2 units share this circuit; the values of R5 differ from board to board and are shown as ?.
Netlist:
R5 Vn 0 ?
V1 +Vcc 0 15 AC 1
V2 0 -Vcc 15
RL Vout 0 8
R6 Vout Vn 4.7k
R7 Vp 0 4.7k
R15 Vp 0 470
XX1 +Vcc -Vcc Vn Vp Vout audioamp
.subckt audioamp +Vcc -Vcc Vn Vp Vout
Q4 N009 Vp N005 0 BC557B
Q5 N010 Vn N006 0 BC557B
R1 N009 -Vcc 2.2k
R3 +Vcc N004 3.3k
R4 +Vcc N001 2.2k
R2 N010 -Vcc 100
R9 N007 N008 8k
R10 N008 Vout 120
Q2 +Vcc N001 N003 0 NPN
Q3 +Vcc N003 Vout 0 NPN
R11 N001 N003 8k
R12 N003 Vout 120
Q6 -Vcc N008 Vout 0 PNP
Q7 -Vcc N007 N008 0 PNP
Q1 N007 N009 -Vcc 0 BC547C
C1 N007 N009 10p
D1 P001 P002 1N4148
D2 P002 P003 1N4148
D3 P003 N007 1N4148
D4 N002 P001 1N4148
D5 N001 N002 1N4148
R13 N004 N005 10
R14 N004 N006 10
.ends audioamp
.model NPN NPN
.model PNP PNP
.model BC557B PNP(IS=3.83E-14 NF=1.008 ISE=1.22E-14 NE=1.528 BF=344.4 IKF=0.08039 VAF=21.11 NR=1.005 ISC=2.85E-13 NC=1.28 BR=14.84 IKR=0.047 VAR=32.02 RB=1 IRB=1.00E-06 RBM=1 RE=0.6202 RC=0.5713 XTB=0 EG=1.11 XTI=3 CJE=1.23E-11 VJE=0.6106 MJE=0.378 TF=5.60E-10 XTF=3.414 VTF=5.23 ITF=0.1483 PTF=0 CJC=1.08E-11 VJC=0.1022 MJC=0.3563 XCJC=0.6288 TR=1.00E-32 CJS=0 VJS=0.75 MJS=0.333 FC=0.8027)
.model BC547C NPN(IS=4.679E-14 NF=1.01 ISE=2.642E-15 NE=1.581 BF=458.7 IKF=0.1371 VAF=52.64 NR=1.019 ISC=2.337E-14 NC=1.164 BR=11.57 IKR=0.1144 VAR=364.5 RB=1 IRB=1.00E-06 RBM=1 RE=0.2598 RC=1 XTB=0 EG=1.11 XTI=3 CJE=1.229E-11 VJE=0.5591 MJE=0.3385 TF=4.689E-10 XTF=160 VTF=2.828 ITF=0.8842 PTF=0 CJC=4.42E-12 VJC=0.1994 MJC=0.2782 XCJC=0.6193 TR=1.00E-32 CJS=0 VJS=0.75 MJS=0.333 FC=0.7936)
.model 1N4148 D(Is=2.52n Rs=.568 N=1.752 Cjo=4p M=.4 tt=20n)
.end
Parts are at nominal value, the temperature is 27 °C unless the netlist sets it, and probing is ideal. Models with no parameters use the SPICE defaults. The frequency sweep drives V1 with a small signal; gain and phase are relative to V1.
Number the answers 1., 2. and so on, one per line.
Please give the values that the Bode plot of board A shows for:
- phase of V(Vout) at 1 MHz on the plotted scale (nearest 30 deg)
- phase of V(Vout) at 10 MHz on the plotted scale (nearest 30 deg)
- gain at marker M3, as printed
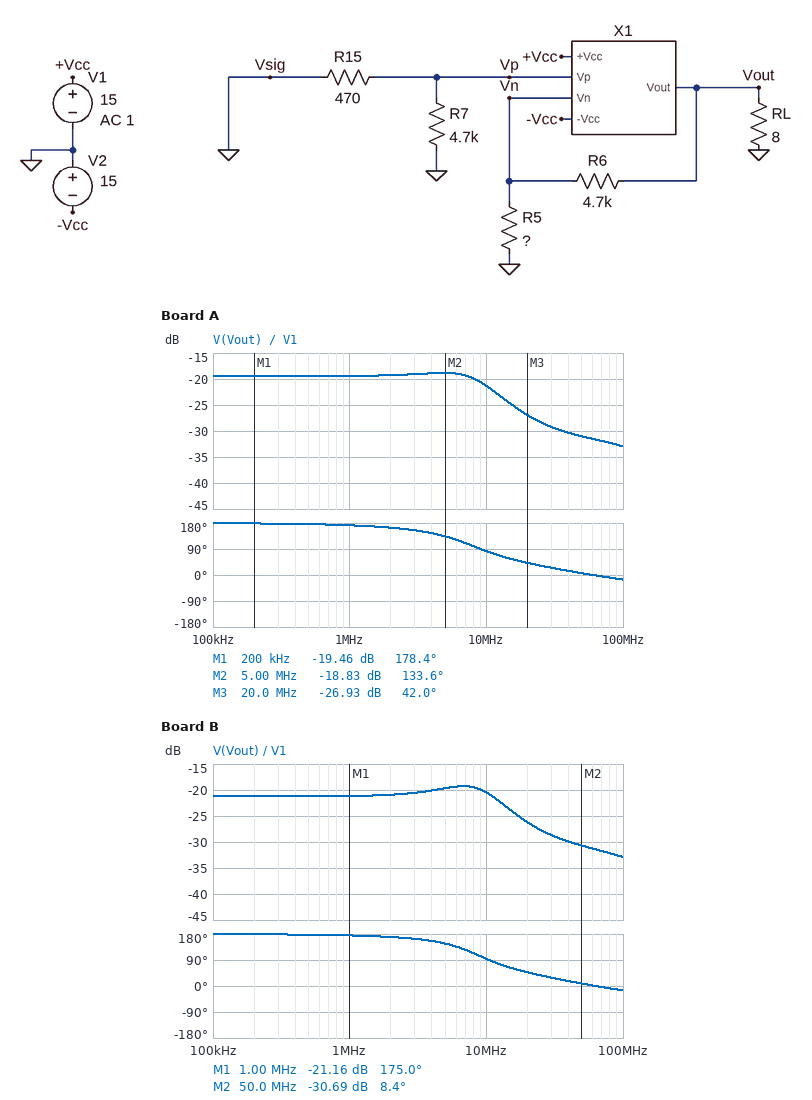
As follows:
1. 180 deg
2. 90 deg
3. -26.93 dB
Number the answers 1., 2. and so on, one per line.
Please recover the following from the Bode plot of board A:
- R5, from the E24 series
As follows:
1. 240 Ω
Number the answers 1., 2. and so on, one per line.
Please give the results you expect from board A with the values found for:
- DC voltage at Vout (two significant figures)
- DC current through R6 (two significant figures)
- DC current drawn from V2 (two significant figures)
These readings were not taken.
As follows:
1. -2.2 V
2. 450 µA
3. 300 mA
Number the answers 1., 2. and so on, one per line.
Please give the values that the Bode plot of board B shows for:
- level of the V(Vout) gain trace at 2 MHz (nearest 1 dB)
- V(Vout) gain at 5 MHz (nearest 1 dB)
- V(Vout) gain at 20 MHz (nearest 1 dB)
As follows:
1. -21 dB
2. -20 dB
3. -26 dB
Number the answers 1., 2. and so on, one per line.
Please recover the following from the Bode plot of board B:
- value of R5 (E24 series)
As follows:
1. 300 Ω
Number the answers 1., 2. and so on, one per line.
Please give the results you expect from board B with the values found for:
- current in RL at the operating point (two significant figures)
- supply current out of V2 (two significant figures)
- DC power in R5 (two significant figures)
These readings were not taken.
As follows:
1. 230 mA
2. 250 mA
3. 38 µW
